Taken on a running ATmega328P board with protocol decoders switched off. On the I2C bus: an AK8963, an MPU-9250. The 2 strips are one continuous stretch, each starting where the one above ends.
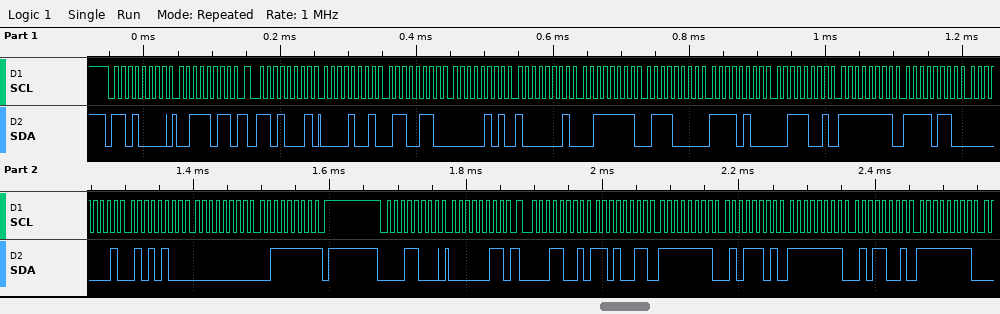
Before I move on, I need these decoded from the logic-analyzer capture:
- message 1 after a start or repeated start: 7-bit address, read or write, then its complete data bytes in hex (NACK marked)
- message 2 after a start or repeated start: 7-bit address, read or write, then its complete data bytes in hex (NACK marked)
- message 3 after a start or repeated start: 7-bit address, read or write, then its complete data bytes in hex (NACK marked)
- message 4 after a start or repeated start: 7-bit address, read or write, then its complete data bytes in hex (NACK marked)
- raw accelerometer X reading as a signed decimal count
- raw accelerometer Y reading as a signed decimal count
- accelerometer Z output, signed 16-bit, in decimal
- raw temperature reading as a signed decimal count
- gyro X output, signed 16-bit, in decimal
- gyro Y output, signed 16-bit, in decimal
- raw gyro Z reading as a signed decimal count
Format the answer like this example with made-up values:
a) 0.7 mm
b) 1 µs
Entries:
a) 0x68 write: 3B
b) 0x68 read: 09 66 05 81 3F 70 F4 39 FF F6 01 54 00 3F NACK
c) 0x0C write: 03
d) 0x0C read: D3 FF 5D FF 59 FF
e) 2406
f) 1409
g) 16240
h) -3015
i) -10
j) 340
k) 63
